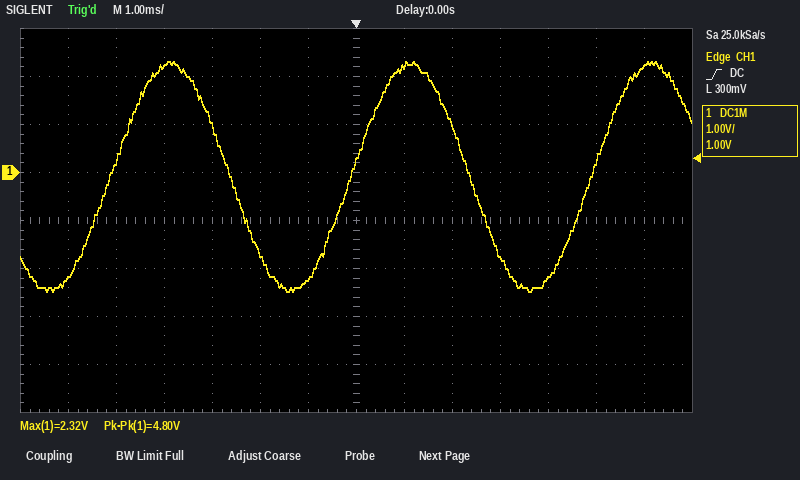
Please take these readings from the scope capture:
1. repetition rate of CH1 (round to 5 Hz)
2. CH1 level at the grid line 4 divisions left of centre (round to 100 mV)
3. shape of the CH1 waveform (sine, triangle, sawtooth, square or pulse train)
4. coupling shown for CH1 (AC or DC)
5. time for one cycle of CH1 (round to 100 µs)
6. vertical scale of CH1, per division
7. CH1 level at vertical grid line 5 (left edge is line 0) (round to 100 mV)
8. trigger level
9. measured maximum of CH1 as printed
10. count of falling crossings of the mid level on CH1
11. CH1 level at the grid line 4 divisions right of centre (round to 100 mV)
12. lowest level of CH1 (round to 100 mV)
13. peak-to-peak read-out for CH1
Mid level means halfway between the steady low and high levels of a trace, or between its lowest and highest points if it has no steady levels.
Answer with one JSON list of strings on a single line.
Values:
["200 Hz", "2.2 V", "sine", "DC", "5.0 ms", "1 V", "-1.7 V", "300 mV", "2.32 V", "2", "-2.2 V", "-2.5 V", "4.80 V"]
